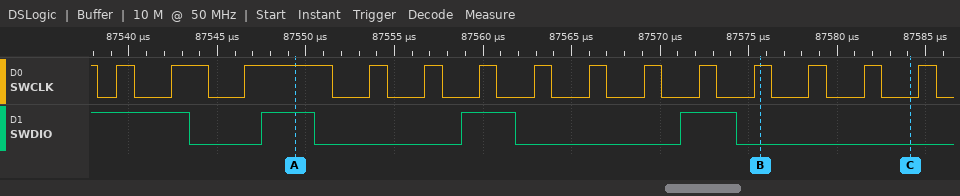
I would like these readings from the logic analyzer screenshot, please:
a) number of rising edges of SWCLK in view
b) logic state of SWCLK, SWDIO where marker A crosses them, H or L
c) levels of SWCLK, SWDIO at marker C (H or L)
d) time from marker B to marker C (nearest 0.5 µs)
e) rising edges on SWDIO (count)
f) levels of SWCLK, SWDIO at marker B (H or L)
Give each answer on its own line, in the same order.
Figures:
14
SWCLK=H, SWDIO=H
SWCLK=L, SWDIO=L
8.5 µs
3
SWCLK=H, SWDIO=L
